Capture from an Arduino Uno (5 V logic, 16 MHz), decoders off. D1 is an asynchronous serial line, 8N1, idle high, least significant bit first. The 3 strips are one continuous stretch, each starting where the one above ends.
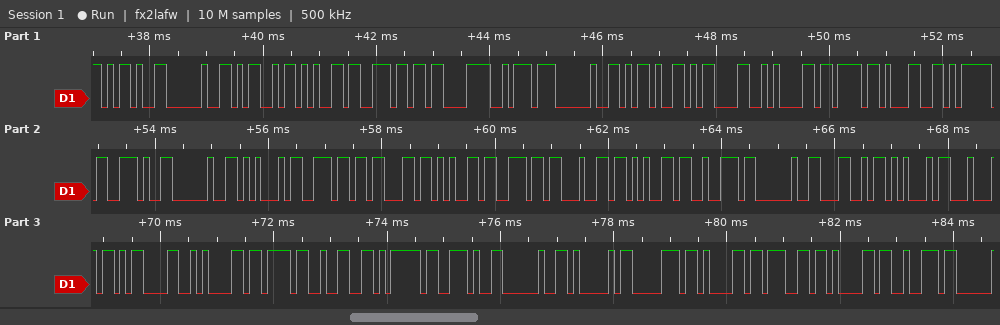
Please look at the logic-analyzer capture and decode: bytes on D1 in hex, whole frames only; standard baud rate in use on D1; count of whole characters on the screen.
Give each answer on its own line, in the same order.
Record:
2D 20 4D 65 6E C3 BA 20 2D 0D 0A 7B 31 7D 2E 20 45 6E 63 65 6E 64 65 72 20 4C 45 44 0D 0A 7B 32 7D 2E 20 41 70 61 67 61 72
9600 baud
41
